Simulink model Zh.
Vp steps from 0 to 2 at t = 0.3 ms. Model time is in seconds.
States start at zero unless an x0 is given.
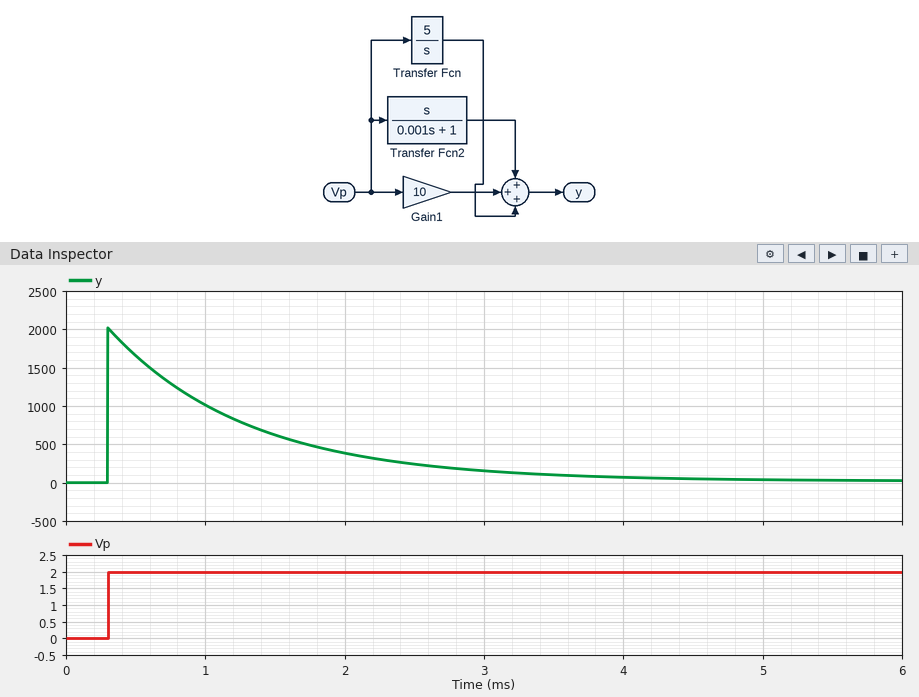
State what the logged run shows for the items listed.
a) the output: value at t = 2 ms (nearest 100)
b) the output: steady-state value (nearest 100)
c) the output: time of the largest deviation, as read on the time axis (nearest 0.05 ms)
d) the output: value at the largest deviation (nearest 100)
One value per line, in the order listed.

400
0
0.30 ms
2000
